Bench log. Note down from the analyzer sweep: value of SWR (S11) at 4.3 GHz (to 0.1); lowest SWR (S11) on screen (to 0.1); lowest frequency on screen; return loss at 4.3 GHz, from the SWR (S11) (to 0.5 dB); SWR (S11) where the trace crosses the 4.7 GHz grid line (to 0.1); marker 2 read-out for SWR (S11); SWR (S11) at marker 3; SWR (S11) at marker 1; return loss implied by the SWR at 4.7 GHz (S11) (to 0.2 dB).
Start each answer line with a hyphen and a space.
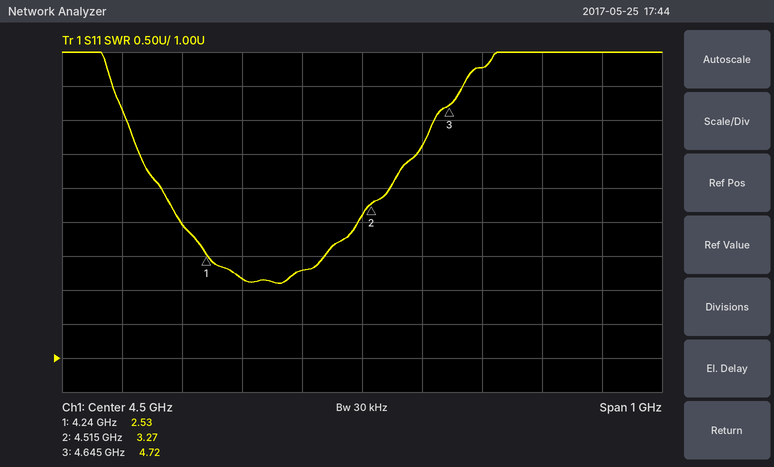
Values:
- 2.2
- 2.1
- 4 GHz
- 8.5 dB
- 5.3
- 3.27
- 4.72
- 2.53
- 3.4 dB
